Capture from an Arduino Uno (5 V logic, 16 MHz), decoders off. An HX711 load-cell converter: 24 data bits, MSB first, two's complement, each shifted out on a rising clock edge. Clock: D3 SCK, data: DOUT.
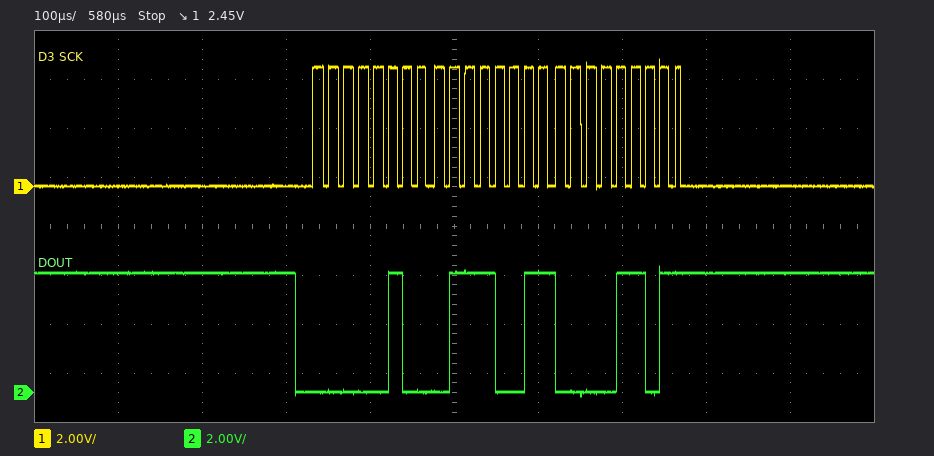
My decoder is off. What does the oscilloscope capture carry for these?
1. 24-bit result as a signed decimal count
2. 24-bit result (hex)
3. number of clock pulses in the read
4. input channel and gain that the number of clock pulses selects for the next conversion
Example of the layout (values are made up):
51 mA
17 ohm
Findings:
291597
0x04730D
25
channel A, gain 128
